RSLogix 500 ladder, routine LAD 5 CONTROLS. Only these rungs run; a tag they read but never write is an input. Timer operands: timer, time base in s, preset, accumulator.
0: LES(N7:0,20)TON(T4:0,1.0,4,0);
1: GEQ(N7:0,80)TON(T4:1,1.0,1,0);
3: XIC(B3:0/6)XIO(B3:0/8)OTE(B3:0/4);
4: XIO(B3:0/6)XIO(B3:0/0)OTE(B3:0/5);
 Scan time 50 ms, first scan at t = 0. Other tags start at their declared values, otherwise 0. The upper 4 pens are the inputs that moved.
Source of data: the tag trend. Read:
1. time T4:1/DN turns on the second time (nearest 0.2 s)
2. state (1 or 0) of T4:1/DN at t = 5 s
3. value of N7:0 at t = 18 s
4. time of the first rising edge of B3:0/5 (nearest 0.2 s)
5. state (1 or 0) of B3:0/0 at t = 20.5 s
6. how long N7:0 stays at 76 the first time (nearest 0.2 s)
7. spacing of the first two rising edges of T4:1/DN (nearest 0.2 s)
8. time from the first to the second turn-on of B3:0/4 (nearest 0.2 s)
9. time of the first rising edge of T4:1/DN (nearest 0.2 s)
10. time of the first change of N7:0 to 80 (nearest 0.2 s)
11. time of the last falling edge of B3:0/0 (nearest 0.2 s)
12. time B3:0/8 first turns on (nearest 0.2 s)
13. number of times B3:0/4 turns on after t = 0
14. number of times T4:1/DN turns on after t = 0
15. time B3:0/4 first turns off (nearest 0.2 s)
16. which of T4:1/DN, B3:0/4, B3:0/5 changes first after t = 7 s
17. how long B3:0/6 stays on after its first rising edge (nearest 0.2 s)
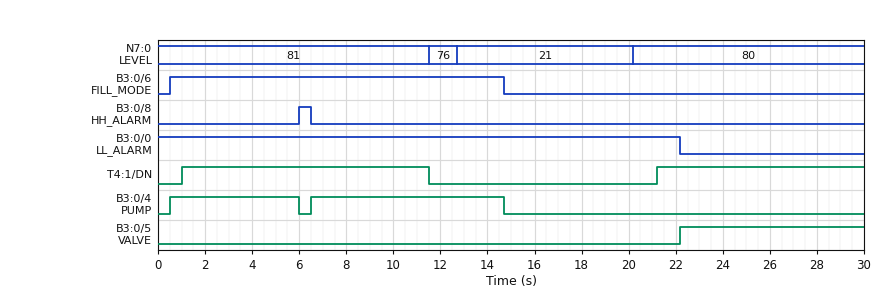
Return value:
21.2 s
1
21
22.2 s
1
1.2 s
20.2 s
6.0 s
1.0 s
20.2 s
22.2 s
6.0 s
2
2
6.0 s
T4:1/DN
14.2 s
